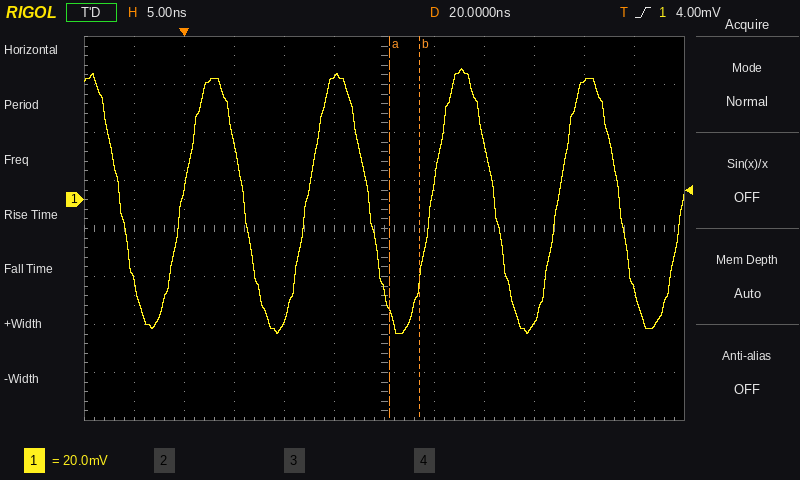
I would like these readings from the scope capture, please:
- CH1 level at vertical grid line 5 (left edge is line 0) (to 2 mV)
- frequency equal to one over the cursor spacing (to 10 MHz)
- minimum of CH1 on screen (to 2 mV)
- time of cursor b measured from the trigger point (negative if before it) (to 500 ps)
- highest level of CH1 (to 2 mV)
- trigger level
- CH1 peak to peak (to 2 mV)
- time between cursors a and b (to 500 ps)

52 mV
330 MHz
-56 mV
+23.5 ns
54 mV
4.00 mV
110 mV
3.0 ns
